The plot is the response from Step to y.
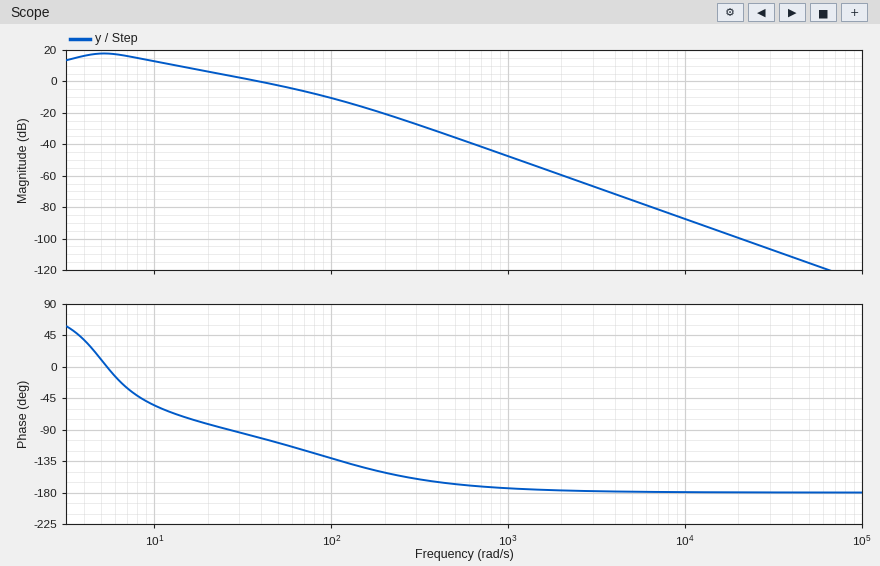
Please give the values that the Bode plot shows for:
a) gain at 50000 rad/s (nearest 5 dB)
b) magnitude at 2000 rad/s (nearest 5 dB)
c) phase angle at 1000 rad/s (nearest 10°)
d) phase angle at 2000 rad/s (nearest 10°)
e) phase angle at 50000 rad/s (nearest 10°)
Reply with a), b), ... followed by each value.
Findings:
a) -115 dB
b) -60 dB
c) -170°
d) -180°
e) -180°
